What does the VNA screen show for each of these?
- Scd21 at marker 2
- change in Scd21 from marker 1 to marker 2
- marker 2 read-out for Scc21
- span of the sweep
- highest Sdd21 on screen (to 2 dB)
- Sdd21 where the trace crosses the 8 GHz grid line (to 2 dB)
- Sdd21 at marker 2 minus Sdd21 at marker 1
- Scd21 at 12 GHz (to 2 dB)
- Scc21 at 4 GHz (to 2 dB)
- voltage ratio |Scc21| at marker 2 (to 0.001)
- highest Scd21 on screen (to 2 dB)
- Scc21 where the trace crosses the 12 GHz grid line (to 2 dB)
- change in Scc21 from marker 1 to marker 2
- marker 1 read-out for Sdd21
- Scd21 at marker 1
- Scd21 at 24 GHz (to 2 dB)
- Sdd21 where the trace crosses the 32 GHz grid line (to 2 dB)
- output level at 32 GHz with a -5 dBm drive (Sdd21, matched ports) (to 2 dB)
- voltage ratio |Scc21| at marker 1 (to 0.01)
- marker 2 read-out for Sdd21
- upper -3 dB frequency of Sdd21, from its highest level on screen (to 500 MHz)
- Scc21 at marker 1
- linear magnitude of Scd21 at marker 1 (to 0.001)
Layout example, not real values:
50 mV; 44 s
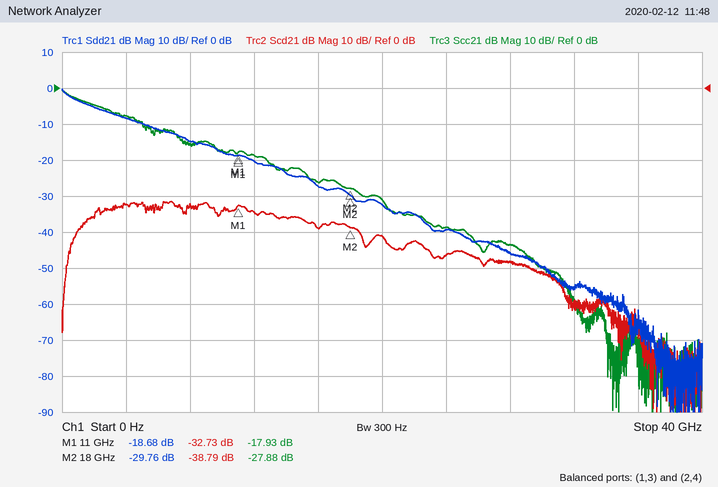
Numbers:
-38.79 dB; -6.06 dB; -27.88 dB; 40 GHz; 0 dB; -14 dB; -11.08 dB; -34 dB; -8 dB; 0.040; -32 dB; -18 dB; -9.95 dB; -18.68 dB; -32.73 dB; -46 dB; -56 dB; -60 dBm; 0.13; -29.76 dB; 1.0 GHz; -17.93 dB; 0.023
